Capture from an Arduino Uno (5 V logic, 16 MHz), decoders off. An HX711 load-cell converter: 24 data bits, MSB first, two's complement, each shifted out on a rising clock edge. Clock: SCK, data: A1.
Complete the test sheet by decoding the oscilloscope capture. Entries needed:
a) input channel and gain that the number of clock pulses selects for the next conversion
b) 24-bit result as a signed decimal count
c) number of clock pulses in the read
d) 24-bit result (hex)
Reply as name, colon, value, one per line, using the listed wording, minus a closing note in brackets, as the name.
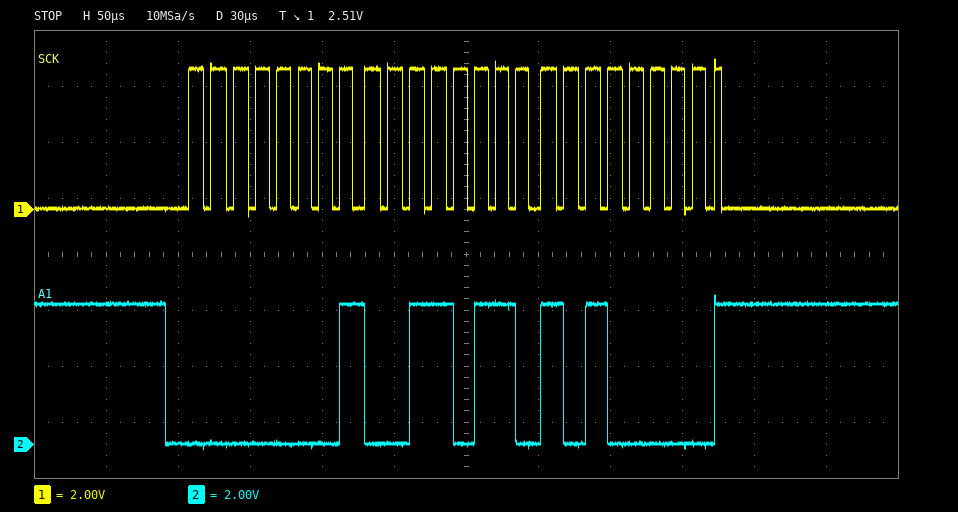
input channel and gain that the number of clock pulses selects for the next conversion: channel A, gain 128
24-bit result as a signed decimal count: 79520
number of clock pulses in the read: 25
24-bit result: 0x0136A0
